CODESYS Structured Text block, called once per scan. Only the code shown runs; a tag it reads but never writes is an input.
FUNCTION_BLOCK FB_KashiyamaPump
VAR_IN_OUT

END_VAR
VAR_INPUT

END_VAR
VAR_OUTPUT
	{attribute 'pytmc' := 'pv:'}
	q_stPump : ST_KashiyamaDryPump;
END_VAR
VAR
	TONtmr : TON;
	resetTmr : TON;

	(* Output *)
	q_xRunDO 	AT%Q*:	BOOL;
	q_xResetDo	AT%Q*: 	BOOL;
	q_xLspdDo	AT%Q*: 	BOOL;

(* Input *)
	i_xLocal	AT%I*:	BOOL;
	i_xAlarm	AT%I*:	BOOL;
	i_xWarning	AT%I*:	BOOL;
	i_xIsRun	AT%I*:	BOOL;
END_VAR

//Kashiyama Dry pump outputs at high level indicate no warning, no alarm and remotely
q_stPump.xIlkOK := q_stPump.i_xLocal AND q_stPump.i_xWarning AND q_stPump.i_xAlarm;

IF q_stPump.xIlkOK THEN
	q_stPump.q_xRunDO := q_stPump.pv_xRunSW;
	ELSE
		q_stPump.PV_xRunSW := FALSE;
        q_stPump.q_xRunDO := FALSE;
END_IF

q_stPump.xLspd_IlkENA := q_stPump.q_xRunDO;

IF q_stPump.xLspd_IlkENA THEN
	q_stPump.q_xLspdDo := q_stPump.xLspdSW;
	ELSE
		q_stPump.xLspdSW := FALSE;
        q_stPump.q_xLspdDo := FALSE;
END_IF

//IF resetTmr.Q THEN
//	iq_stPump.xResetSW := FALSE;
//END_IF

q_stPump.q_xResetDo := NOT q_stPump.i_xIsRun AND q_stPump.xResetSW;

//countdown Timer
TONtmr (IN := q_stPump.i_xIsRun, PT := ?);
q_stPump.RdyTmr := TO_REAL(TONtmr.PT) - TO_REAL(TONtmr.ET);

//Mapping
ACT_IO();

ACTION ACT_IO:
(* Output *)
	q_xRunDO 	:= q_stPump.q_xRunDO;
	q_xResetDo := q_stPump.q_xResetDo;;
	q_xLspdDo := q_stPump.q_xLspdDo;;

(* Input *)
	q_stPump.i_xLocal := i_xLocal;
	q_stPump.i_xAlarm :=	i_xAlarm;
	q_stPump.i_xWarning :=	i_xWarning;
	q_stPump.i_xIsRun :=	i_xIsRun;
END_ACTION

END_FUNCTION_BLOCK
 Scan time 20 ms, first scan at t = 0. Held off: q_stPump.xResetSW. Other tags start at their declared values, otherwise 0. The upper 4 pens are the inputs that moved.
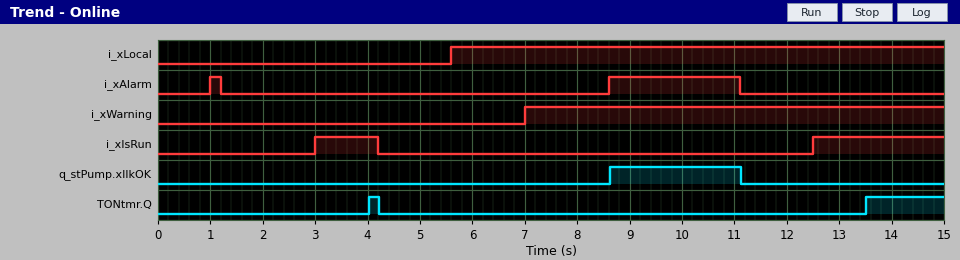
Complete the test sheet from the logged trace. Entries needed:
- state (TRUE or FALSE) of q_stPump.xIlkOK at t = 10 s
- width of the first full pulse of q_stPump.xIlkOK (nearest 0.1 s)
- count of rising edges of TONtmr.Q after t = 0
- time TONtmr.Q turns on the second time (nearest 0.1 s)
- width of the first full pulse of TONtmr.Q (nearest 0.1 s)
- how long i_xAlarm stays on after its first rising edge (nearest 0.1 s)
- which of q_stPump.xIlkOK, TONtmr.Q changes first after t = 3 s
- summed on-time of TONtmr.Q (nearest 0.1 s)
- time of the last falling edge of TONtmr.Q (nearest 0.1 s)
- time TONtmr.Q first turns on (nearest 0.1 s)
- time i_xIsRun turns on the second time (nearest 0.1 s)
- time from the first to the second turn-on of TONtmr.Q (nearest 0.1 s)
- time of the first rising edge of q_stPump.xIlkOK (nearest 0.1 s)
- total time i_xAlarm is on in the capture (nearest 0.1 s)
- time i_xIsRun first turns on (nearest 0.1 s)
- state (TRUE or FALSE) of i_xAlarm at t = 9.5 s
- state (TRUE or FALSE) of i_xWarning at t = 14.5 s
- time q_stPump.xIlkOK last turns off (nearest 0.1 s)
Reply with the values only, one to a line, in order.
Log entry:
TRUE
2.5 s
2
13.5 s
0.2 s
0.2 s
TONtmr.Q
1.7 s
4.2 s
4.0 s
12.5 s
9.5 s
8.6 s
2.7 s
3.0 s
TRUE
TRUE
11.1 s
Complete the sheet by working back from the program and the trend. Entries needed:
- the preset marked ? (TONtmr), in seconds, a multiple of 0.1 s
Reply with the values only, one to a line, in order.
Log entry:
1.0 s
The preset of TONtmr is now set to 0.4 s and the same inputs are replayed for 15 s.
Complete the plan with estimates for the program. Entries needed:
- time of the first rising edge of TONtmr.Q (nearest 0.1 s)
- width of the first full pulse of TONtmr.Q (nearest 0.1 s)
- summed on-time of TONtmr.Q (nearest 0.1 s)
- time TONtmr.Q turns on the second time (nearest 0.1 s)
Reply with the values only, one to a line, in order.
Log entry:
3.4 s
0.8 s
2.9 s
12.9 s
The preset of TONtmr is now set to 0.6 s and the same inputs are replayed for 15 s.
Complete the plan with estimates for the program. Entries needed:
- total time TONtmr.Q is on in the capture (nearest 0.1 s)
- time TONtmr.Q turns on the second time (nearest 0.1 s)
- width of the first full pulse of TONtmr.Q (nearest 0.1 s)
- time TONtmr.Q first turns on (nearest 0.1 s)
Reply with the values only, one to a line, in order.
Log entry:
2.5 s
13.1 s
0.6 s
3.6 s
